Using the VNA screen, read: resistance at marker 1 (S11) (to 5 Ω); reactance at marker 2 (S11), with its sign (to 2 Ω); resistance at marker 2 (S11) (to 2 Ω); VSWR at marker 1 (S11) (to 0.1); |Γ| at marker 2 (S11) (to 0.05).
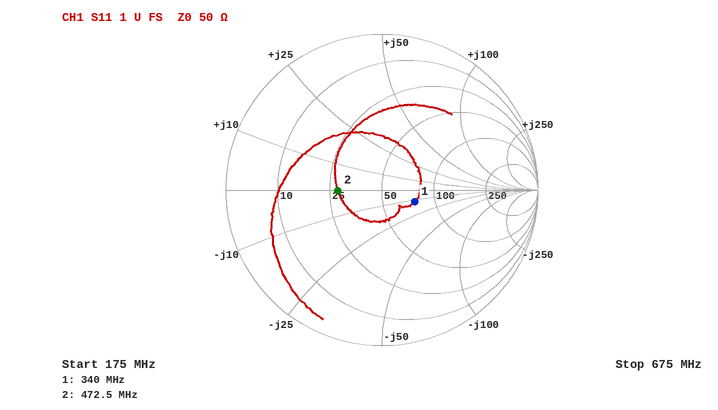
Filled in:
75 Ω
0 Ω
28 Ω
1.6
0.30
